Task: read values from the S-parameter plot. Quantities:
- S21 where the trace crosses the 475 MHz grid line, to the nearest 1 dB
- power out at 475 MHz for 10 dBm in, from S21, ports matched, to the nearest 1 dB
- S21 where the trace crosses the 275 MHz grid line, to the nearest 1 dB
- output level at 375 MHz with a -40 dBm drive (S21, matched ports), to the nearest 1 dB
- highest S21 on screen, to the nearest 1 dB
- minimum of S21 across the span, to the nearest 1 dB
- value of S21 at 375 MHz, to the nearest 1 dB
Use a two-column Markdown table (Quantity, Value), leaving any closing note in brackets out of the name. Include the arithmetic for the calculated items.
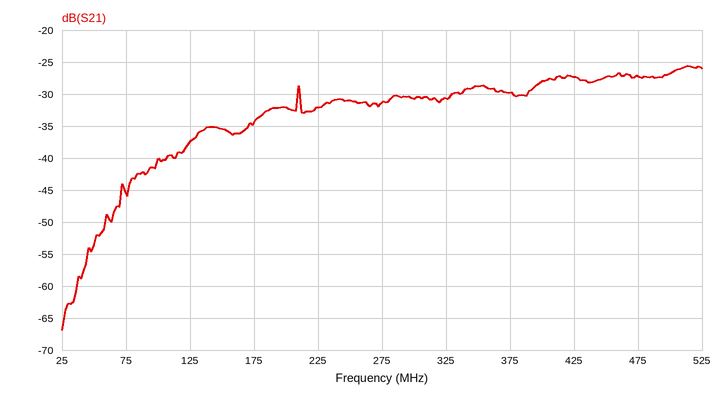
| Quantity | Value |
|---|---|
| S21 where the trace crosses the 475 MHz grid line, to the nearest 1 dB | -27 dB |
| power out at 475 MHz for 10 dBm in, from S21, ports matched, to the nearest 1 dB | 10 dBm + (-27 dB) = -17 dBm |
| S21 where the trace crosses the 275 MHz grid line, to the nearest 1 dB | -31 dB |
| output level at 375 MHz with a -40 dBm drive (S21, matched ports), to the nearest 1 dB | -40 dBm + (-30 dB) = -70 dBm |
| highest S21 on screen, to the nearest 1 dB | -26 dB |
| minimum of S21 across the span, to the nearest 1 dB | -67 dB |
| value of S21 at 375 MHz, to the nearest 1 dB | -30 dB |
